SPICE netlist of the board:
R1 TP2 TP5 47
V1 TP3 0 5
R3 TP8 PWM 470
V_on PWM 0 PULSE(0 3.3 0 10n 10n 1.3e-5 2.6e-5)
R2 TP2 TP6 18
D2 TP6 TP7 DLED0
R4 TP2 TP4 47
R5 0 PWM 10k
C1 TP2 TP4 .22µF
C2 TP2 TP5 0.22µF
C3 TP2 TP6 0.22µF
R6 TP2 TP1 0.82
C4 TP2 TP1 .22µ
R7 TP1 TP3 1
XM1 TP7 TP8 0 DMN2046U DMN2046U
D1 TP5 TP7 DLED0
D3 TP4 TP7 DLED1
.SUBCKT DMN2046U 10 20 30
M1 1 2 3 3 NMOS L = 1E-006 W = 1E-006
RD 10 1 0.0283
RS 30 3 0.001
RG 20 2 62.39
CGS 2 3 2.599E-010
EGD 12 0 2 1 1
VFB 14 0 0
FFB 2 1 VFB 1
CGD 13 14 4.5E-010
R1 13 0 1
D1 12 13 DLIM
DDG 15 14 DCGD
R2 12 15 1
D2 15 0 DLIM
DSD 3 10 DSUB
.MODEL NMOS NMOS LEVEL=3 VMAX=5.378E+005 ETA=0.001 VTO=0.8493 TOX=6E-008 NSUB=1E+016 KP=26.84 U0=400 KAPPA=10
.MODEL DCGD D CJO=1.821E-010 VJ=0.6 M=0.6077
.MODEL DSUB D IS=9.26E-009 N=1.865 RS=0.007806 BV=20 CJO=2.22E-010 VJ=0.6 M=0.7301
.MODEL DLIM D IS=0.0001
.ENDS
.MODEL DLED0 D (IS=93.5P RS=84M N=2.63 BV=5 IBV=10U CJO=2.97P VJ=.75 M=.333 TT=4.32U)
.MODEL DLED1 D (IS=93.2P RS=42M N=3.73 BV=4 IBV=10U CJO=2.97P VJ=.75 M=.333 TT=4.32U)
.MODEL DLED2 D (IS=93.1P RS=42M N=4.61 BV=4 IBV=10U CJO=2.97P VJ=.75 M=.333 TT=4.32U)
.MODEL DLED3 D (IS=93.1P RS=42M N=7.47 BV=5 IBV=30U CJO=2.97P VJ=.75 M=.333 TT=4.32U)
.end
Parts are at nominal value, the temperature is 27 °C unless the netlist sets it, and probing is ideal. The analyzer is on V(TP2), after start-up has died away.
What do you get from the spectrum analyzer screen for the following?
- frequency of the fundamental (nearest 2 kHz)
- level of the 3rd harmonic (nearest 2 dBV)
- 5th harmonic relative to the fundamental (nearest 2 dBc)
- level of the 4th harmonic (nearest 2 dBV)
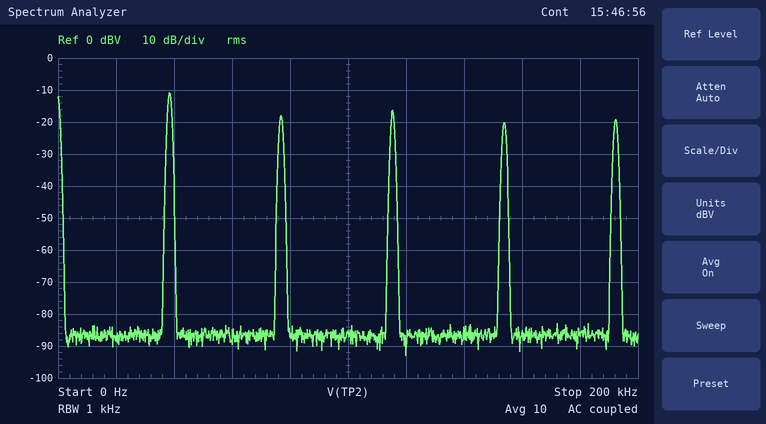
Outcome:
38 kHz
-16 dBV
-8 dBc
-20 dBV
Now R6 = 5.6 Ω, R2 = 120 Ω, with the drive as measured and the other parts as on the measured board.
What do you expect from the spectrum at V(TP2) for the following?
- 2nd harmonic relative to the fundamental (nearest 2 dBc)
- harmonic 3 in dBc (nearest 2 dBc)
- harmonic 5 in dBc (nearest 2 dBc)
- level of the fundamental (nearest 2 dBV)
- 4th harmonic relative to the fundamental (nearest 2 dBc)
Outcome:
-10 dBc
-10 dBc
-14 dBc
-6 dBV
-14 dBc
